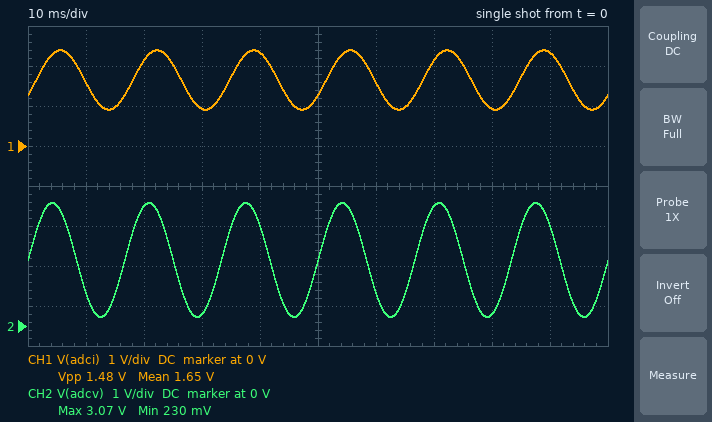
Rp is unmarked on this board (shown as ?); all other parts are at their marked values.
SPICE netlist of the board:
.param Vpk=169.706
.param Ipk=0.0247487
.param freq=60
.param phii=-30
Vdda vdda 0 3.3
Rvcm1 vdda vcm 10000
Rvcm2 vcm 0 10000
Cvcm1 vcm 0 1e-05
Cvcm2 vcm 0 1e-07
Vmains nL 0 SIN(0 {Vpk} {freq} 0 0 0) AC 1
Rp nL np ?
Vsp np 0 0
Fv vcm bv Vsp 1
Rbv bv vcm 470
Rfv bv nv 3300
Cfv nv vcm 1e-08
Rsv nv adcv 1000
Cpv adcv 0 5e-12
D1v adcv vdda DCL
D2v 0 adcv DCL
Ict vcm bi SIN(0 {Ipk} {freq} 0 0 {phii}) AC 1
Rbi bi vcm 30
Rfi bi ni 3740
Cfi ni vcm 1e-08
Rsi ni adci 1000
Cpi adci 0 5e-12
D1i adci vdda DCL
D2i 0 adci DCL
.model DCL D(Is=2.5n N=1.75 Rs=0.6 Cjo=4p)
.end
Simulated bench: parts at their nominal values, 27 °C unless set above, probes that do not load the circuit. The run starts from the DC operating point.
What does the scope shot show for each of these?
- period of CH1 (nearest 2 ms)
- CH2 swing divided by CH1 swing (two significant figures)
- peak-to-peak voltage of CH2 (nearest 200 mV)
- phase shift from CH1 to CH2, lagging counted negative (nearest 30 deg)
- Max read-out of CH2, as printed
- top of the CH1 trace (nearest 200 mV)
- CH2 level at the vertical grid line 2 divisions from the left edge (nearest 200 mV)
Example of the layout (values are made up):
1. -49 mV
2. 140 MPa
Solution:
1. 16 ms
2. 1.9
3. 2.8 V
4. 30 deg
5. 3.07 V
6. 2.4 V
7. 3.0 V
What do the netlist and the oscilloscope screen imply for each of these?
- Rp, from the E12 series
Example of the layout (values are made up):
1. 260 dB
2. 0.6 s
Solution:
1. 56 kΩ
